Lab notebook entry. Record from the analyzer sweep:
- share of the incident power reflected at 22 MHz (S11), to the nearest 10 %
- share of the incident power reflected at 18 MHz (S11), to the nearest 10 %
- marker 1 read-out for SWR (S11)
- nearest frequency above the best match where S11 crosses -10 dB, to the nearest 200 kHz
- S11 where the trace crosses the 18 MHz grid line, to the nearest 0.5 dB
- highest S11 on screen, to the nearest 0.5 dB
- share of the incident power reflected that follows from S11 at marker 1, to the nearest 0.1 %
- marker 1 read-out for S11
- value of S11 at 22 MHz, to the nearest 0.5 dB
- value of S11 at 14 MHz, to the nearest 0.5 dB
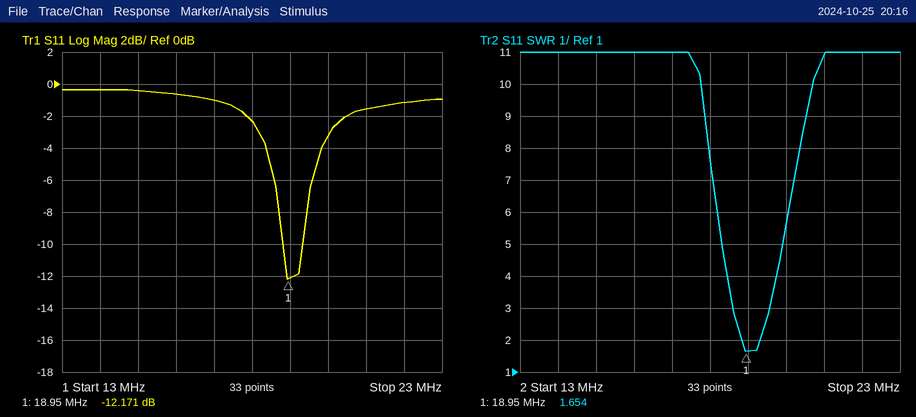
80 %
60 %
1.654
19.4 MHz
-2.5 dB
-0.5 dB
6.1 %
-12.171 dB
-1.0 dB
-0.5 dB
